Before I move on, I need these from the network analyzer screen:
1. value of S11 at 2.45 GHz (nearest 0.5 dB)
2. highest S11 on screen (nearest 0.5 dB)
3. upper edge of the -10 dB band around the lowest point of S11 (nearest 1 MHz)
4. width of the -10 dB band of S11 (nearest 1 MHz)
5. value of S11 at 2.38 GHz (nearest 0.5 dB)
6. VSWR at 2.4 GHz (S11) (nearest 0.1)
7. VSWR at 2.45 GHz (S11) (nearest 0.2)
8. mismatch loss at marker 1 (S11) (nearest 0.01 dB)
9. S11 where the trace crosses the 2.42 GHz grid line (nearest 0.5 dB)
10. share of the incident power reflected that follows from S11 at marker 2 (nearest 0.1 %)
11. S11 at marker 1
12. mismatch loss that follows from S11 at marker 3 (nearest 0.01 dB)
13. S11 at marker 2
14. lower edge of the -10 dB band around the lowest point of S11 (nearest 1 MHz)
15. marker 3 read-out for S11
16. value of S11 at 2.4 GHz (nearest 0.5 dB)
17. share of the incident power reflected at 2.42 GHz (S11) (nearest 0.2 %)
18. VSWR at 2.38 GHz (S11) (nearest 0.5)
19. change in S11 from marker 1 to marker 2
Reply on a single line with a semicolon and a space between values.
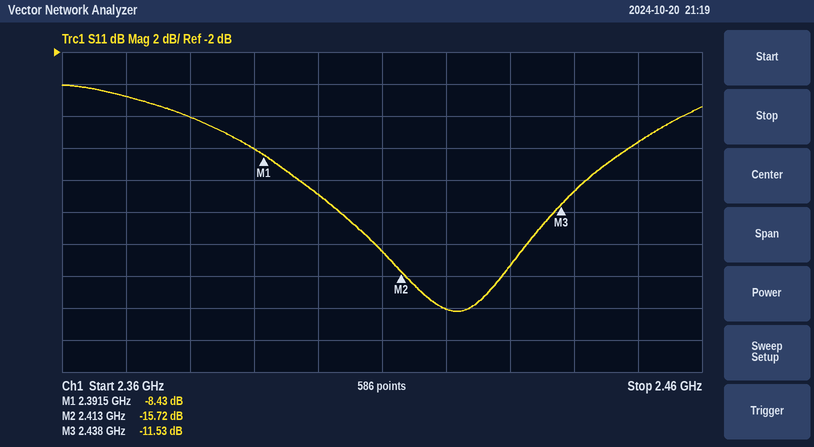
-7.5 dB; -4.0 dB; 2.442 GHz; 45 MHz; -6.0 dB; 1.8; 2.4; 0.67 dB; -18.0 dB; 2.7 %; -8.43 dB; 0.32 dB; -15.72 dB; 2.397 GHz; -11.53 dB; -11.0 dB; 1.6 %; 3.0; -7.29 dB
